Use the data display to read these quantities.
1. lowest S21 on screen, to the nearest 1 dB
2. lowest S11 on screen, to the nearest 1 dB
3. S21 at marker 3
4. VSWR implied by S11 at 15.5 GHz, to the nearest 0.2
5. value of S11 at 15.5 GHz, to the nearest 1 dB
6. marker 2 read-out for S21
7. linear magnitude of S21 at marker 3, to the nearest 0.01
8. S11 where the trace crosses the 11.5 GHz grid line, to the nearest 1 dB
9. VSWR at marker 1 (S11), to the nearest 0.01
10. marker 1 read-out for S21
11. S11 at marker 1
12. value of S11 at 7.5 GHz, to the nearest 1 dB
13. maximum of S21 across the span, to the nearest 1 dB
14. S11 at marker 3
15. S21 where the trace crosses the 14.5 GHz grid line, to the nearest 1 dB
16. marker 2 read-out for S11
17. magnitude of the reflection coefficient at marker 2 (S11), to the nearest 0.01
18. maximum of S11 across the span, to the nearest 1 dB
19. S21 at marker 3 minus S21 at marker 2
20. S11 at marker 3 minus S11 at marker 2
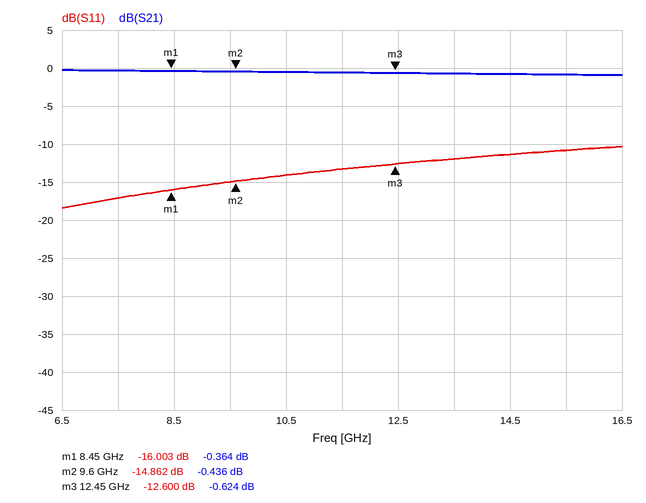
-1 dB
-18 dB
-0.624 dB
1.8
-11 dB
-0.436 dB
0.93
-13 dB
1.38
-0.364 dB
-16.003 dB
-17 dB
0 dB
-12.600 dB
-1 dB
-14.862 dB
0.18
-10 dB
-0.188 dB
2.262 dB
